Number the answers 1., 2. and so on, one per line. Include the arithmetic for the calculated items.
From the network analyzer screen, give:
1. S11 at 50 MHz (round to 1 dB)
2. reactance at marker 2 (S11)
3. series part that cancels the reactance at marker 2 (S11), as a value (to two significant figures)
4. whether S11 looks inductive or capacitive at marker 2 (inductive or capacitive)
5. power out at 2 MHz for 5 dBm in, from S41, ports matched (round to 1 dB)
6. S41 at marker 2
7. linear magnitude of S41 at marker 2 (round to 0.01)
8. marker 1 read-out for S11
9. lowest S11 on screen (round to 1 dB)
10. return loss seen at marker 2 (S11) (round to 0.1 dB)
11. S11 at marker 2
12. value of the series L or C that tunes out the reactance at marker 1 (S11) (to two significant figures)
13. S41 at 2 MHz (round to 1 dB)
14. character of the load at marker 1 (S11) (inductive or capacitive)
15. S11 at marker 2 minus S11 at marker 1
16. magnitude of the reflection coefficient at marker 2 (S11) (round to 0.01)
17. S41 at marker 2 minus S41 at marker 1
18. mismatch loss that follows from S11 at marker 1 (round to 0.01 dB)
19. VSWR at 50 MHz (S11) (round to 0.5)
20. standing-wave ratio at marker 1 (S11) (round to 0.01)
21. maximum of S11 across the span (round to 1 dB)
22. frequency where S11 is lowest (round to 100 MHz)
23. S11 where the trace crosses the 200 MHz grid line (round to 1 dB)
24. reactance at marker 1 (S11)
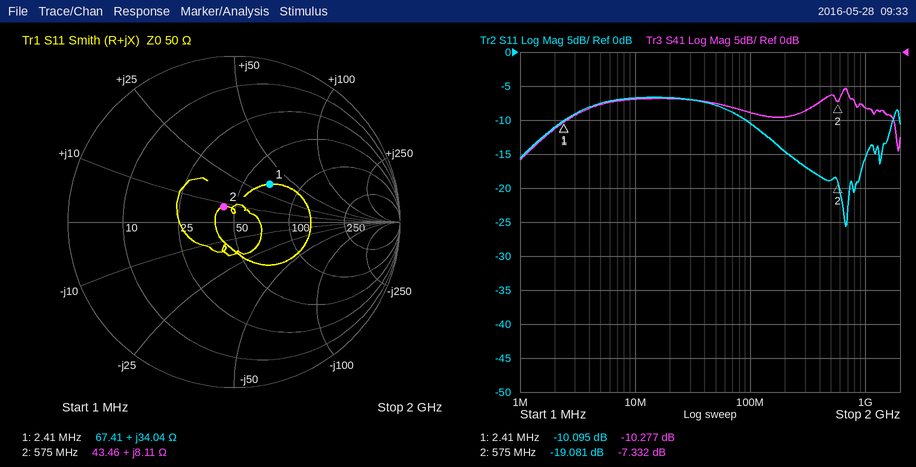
1. -8 dB
2. +8.11 Ω
3. C = 1/(2π × 575 MHz × 8.11 Ω) ≈ 34 pF
4. inductive
5. 5 dBm + (-11 dB) = -6 dBm
6. -7.332 dB
7. 10^(-7.332/20) ≈ 0.43
8. -10.095 dB
9. -26 dB
10. 19.1 dB
11. -19.081 dB
12. C = 1/(2π × 2.41 MHz × 34.04 Ω) ≈ 1.9 nF
13. -11 dB
14. inductive
15. -19.081 − (-10.095) = -8.986 dB
16. 10^(-19.081/20) ≈ 0.11
17. -7.332 − (-10.277) = 2.945 dB
18. −10 log10(1 − 10^(-10.095/10)) ≈ 0.45 dB
19. |Γ| = 10^(-8/20) = 0.3981; VSWR = (1 + 0.3981)/(1 − 0.3981) ≈ 2.32, so 2.5 to the nearest 0.5
20. 1.91
21. -7 dB
22. 700 MHz
23. -15 dB
24. +34.04 Ω
